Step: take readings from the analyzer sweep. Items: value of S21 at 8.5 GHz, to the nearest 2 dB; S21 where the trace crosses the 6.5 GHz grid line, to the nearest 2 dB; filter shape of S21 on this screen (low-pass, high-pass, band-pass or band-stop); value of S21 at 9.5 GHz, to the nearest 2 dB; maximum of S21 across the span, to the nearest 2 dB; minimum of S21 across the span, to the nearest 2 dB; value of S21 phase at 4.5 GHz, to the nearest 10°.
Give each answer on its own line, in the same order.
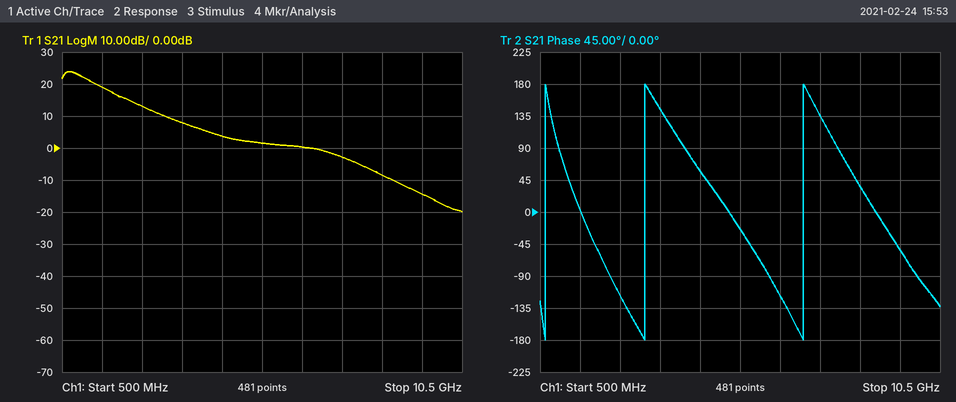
-8 dB
0 dB
low-pass
-14 dB
24 dB
-20 dB
60°
